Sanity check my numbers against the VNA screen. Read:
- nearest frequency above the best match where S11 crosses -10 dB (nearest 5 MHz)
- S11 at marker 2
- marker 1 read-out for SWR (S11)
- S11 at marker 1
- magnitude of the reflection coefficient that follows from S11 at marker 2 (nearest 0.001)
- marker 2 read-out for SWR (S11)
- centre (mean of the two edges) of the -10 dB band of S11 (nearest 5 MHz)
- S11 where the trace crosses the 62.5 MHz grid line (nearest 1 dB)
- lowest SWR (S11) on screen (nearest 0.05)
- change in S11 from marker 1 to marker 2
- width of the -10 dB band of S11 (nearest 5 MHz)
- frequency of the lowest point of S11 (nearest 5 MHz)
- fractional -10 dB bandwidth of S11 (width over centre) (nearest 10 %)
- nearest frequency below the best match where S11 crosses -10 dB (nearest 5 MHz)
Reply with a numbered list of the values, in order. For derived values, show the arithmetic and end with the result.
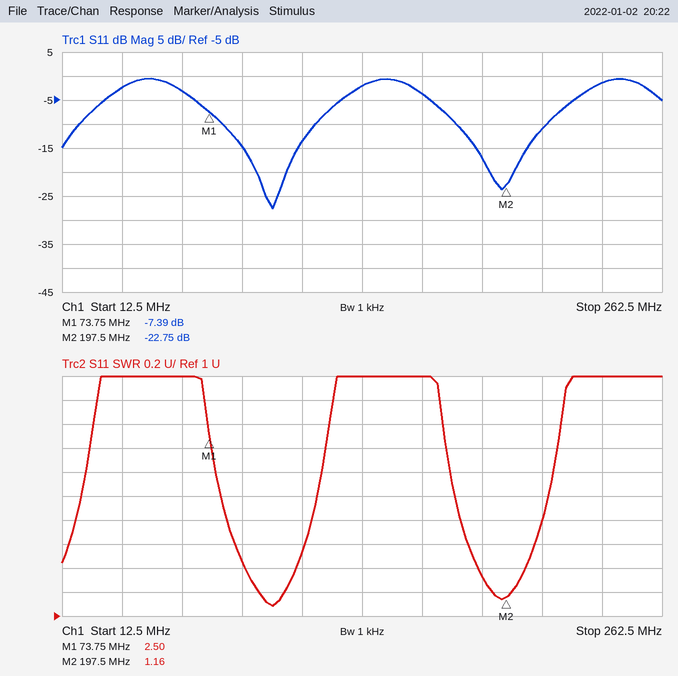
1. 120 MHz
2. -22.75 dB
3. 2.50
4. -7.39 dB
5. 10^(-22.75/20) ≈ 0.073
6. 1.16
7. 100 MHz
8. -3 dB
9. 1.10
10. -22.75 − (-7.39) = -15.36 dB
11. 120 MHz − 80 MHz = 40 MHz
12. 100 MHz
13. 40 MHz / 100 MHz ≈ 40 %
14. 80 MHz
